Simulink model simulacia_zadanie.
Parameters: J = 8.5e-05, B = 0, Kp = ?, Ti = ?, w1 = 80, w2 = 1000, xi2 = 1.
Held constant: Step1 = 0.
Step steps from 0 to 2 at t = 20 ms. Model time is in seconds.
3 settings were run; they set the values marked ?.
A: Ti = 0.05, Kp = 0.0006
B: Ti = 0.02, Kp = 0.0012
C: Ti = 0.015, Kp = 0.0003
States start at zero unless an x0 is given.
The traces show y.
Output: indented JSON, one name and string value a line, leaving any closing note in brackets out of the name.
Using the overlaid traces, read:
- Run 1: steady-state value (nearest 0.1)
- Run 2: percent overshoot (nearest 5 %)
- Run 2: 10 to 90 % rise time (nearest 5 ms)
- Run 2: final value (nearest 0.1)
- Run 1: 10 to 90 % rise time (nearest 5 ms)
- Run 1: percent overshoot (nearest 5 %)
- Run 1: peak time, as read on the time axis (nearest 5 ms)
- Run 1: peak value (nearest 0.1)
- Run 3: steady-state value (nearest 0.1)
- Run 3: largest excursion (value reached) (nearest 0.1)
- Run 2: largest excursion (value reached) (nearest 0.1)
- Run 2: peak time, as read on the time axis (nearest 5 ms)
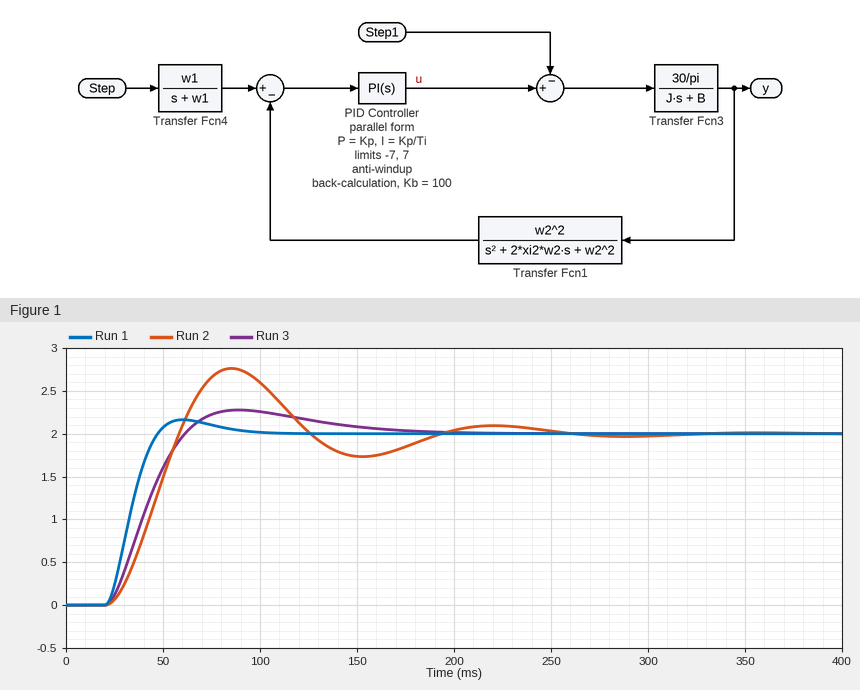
{
  "Run 1: steady-state value": "2.0",
  "Run 2: percent overshoot": "40 %",
  "Run 2: 10 to 90 % rise time": "25 ms",
  "Run 2: final value": "2.0",
  "Run 1: 10 to 90 % rise time": "20 ms",
  "Run 1: percent overshoot": "10 %",
  "Run 1: peak time, as read on the time axis": "60 ms",
  "Run 1: peak value": "2.2",
  "Run 3: steady-state value": "2.0",
  "Run 3: largest excursion (value reached)": "2.3",
  "Run 2: largest excursion (value reached)": "2.8",
  "Run 2: peak time, as read on the time axis": "85 ms"
}
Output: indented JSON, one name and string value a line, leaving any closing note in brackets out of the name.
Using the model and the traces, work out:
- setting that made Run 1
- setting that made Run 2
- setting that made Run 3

{
  "setting that made Run 1": "B",
  "setting that made Run 2": "C",
  "setting that made Run 3": "A"
}
